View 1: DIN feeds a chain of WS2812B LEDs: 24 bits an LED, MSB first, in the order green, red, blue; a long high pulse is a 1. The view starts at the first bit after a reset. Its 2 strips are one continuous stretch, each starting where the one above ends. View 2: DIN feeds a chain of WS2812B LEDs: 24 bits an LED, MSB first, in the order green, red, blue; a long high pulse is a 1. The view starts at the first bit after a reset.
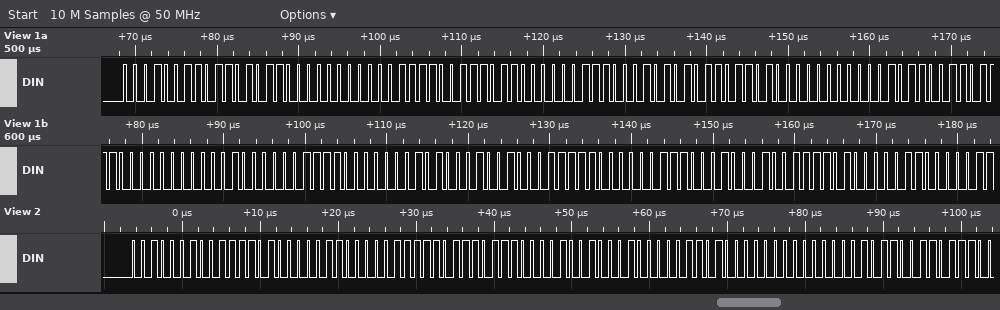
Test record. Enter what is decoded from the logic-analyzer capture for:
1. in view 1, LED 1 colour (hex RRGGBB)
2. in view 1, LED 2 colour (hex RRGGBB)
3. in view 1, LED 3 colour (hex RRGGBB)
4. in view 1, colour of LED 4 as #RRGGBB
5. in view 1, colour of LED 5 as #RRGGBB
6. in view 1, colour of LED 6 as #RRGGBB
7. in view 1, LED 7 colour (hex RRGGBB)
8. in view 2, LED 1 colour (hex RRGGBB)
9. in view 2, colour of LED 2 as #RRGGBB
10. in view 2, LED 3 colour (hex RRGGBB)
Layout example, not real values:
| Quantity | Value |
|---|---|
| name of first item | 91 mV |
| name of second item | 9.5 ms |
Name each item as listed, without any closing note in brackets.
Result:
| Quantity | Value |
|---|---|
| in view 1, LED 1 colour | #6B1300 |
| in view 1, LED 2 colour | #761E07 |
| in view 1, LED 3 colour | #6D1500 |
| in view 1, colour of LED 4 as #RRGGBB | #6E1600 |
| in view 1, colour of LED 5 as #RRGGBB | #78200A |
| in view 1, colour of LED 6 as #RRGGBB | #7C240E |
| in view 1, LED 7 colour | #7A220C |
| in view 2, LED 1 colour | #7A220C |
| in view 2, colour of LED 2 as #RRGGBB | #771F09 |
| in view 2, LED 3 colour | #681000 |
